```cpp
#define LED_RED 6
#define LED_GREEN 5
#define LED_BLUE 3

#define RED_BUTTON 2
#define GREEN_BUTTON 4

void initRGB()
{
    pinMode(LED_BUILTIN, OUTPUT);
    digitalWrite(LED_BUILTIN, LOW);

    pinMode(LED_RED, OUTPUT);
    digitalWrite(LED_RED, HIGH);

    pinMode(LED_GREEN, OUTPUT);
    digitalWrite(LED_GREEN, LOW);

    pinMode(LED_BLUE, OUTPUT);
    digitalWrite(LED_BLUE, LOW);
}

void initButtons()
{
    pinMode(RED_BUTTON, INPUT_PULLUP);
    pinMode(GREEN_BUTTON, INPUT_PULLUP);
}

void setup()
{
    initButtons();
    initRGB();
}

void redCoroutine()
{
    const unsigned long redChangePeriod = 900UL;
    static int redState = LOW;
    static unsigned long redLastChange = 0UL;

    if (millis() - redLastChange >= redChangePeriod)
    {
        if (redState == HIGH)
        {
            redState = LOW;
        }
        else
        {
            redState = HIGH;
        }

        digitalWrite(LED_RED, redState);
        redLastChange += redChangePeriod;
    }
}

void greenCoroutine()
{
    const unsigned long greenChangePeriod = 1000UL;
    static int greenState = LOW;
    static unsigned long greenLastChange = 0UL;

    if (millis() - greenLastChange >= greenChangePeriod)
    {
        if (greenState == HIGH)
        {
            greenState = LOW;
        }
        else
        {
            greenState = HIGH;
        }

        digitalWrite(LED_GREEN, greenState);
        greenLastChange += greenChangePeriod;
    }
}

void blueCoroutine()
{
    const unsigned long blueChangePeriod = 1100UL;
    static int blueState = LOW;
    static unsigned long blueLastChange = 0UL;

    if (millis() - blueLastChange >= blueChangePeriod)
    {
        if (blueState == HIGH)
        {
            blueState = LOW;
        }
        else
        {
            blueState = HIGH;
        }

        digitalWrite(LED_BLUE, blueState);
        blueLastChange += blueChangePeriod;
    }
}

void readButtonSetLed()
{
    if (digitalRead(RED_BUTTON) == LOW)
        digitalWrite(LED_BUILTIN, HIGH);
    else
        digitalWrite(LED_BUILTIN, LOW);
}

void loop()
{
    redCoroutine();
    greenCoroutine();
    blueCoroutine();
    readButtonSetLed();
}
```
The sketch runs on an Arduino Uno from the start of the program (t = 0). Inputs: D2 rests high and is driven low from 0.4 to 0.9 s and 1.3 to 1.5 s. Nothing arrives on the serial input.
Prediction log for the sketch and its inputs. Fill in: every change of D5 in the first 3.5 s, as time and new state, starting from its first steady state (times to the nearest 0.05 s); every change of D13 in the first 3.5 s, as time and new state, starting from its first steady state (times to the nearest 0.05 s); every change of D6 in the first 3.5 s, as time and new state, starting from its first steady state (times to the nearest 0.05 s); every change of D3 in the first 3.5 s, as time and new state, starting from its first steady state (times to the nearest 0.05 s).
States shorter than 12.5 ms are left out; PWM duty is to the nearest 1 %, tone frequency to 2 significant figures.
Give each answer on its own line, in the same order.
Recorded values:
0 s low; 1 s high; 2 s low; 3 s high
0 s low; 0.4 s high; 0.9 s low; 1.3 s high; 1.5 s low
0 s high; 1.8 s low; 2.7 s high
0 s low; 1.1 s high; 2.2 s low; 3.3 s high
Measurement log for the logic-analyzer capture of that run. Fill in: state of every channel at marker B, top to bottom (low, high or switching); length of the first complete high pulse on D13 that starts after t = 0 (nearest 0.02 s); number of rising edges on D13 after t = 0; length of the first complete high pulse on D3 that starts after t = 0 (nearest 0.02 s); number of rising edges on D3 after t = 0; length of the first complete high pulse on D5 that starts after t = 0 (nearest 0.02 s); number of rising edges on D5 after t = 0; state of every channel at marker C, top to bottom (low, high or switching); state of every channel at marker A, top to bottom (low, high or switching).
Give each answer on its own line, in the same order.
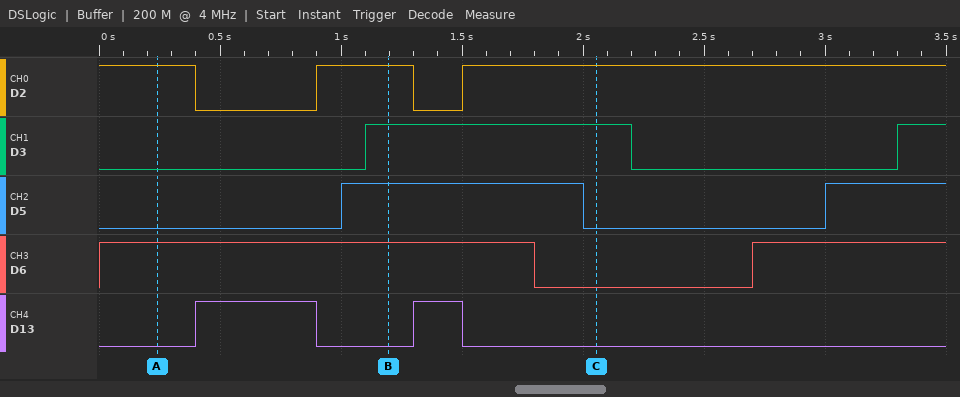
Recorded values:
D2 high, D3 high, D5 high, D6 high, D13 low
0.50 s
2
1.10 s
2
1.00 s
2
D2 high, D3 high, D5 low, D6 low, D13 low
D2 high, D3 low, D5 low, D6 high, D13 low
